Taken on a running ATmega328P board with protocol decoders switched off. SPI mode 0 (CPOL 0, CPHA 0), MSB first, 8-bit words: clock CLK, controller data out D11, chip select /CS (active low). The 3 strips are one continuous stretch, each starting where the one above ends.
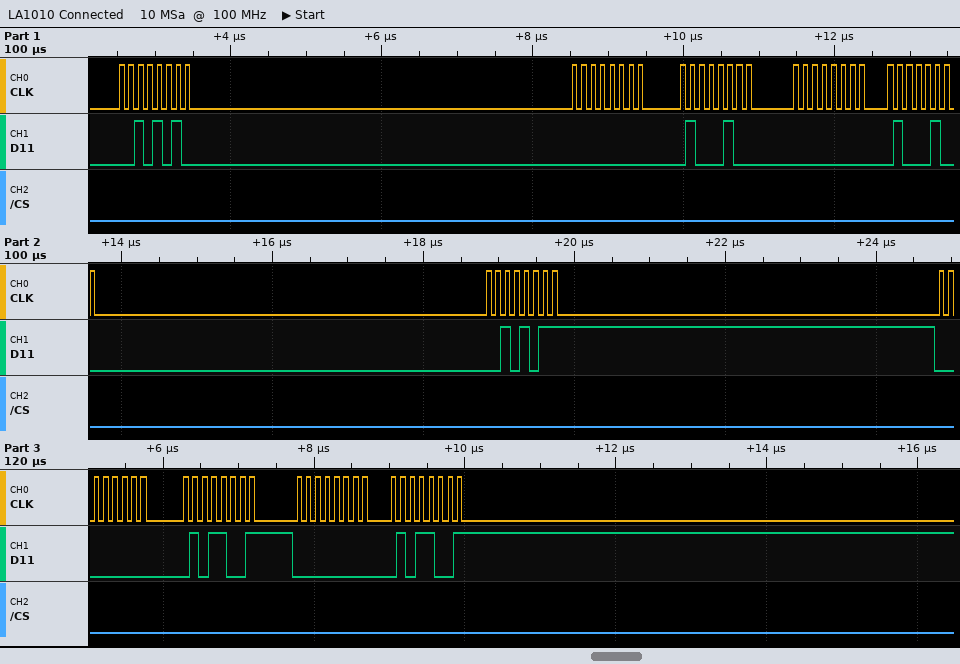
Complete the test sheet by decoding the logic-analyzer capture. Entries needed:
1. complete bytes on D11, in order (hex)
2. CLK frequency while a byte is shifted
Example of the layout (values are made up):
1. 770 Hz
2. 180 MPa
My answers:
1. 2A 00 44 00 44 2B 00 59 00 59
2. 8 MHz
